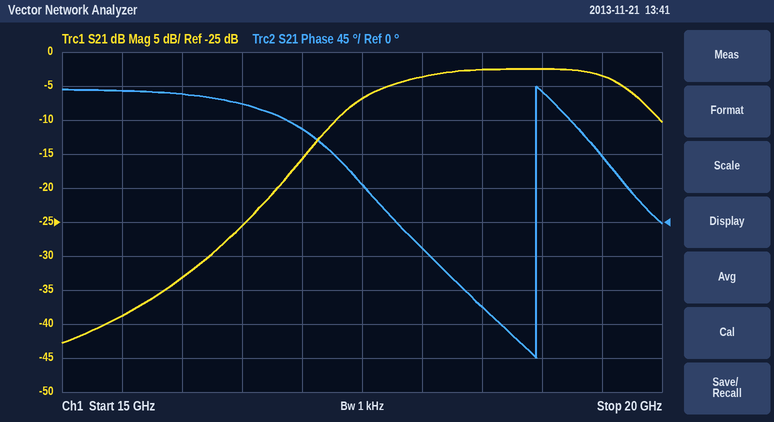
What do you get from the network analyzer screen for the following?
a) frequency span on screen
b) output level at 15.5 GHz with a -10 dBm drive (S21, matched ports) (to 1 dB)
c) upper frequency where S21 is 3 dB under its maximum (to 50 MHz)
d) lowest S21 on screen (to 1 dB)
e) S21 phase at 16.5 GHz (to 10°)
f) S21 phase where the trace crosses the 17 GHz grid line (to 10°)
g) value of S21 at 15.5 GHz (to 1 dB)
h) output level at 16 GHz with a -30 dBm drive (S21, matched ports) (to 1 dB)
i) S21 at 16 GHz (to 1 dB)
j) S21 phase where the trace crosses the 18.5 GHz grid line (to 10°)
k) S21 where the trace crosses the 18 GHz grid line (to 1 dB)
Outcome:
5 GHz
-49 dBm
19.70 GHz
-43 dB
160°
120°
-39 dB
-63 dBm
-33 dB
-110°
-4 dB
